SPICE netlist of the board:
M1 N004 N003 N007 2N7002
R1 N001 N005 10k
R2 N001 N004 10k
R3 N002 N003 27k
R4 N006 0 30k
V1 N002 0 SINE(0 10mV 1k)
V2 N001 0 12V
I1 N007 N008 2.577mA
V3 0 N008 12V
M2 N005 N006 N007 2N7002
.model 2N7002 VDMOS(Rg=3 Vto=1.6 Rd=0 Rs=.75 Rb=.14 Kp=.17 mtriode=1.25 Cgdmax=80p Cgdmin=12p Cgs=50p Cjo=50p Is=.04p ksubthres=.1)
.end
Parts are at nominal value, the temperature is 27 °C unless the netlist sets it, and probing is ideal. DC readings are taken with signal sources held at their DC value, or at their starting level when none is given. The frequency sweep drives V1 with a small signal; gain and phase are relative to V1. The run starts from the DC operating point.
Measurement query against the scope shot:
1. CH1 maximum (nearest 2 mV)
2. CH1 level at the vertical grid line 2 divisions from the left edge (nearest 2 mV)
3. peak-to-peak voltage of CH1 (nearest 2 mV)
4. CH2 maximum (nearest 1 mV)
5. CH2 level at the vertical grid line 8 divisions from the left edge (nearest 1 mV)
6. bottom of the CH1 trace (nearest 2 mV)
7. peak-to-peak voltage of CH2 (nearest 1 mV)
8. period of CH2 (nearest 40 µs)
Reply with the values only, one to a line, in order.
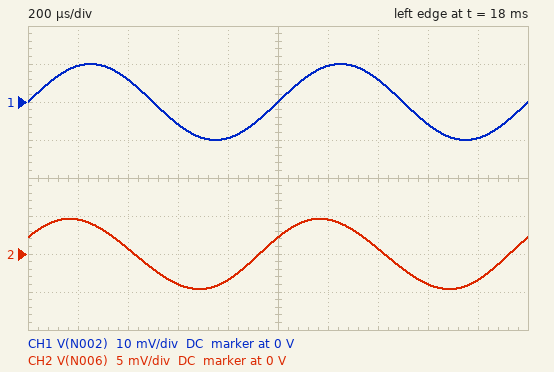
10 mV
6 mV
20 mV
5 mV
-4 mV
-10 mV
9 mV
1.00 ms
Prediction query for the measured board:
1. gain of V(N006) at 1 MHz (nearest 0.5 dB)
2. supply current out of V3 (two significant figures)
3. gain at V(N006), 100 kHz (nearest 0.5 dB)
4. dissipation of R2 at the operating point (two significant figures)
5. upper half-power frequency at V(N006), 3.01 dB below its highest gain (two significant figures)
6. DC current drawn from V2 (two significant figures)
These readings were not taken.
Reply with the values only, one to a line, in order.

-17.0 dB
2.6 mA
-11.0 dB
17 mW
63 kHz
2.6 mA
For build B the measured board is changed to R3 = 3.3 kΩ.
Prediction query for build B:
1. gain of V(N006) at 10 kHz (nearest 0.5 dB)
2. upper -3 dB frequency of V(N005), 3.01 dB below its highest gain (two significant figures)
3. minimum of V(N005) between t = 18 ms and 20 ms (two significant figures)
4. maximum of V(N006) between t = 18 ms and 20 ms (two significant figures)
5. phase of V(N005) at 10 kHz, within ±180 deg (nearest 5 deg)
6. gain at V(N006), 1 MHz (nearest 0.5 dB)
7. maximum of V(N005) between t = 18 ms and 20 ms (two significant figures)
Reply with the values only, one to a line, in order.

-1.0 dB
880 Hz
-1.4 V
6.7 mV
-80 deg
-5.0 dB
-390 mV
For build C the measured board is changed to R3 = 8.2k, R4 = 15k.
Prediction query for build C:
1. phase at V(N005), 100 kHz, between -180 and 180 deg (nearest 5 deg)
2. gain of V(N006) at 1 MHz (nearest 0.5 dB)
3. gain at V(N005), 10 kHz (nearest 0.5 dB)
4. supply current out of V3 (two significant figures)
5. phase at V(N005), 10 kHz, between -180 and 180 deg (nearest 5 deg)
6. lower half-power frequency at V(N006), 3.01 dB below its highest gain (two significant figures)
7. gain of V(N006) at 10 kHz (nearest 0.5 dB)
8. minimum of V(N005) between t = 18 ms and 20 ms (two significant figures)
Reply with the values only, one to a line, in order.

-75 deg
-10.0 dB
19.5 dB
2.6 mA
-80 deg
1.2 kHz
-4.0 dB
-1.5 V
